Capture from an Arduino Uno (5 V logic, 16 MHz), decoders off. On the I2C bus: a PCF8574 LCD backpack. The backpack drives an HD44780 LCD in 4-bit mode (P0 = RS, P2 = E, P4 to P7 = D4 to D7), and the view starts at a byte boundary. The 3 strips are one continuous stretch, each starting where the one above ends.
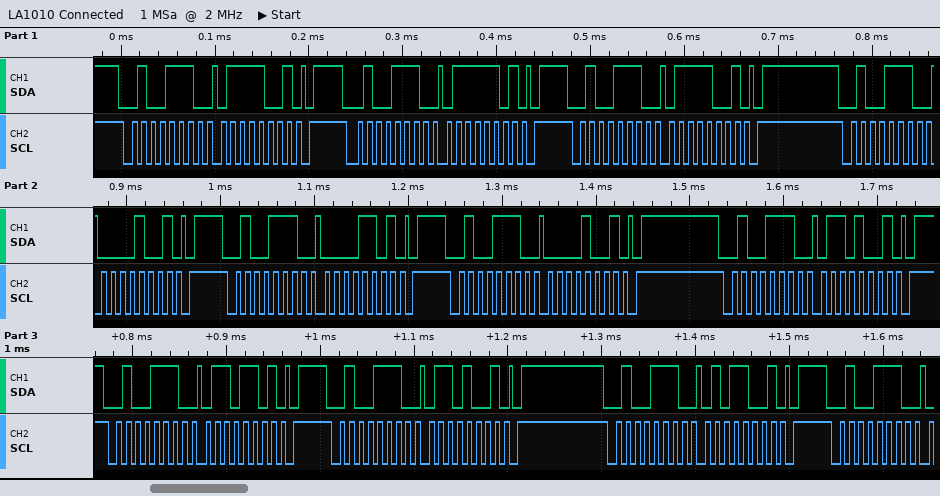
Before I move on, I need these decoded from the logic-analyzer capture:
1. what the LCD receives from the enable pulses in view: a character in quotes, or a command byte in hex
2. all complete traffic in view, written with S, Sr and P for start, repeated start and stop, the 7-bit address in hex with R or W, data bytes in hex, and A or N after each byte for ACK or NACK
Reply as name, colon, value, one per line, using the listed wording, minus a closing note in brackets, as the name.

what the LCD receives from the enable pulses in view: a character in quotes, or a command byte in hex: 'p'
all complete traffic in view, written with S, Sr and P for start, repeated start and stop, the 7-bit address in hex with R or W, data bytes in hex, and A or N after each byte for ACK or NACK: S 27W A 79 A P S 27W A 7D A P S 27W A 79 A P S 27W A 09 A P S 27W A 0D A P S 27W A 09 A P S 27W A 69 A P S 27W A 6D A P S 27W A 69 A P S 27W A 59 A P S 27W A
